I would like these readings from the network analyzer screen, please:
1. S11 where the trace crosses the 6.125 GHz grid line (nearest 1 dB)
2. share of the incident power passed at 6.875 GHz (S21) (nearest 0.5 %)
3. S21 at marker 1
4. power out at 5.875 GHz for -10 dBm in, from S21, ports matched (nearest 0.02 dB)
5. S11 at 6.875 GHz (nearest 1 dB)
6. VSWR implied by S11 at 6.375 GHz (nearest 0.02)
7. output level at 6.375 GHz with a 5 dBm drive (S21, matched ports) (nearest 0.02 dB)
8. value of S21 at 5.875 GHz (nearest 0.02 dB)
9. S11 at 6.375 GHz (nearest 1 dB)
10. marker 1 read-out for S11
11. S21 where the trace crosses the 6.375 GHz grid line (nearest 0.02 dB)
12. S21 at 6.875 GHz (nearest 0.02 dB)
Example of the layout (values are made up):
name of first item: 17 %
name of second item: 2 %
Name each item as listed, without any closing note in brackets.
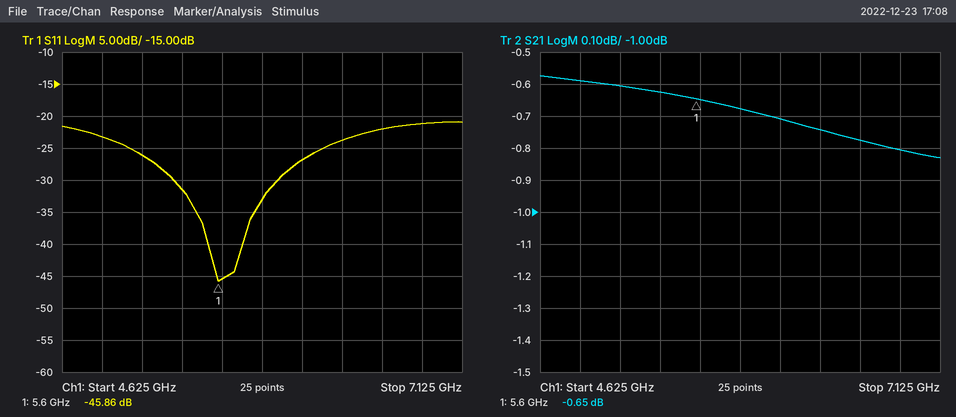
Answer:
S11 where the trace crosses the 6.125 GHz grid line: -27 dB
share of the incident power passed at 6.875 GHz (S21): 83.0 %
S21 at marker 1: -0.65 dB
power out at 5.875 GHz for -10 dBm in, from S21, ports matched: -10.68 dBm
S11 at 6.875 GHz: -21 dB
VSWR implied by S11 at 6.375 GHz: 1.14
output level at 6.375 GHz with a 5 dBm drive (S21, matched ports): 4.26 dBm
value of S21 at 5.875 GHz: -0.68 dB
S11 at 6.375 GHz: -24 dB
marker 1 read-out for S11: -45.86 dB
S21 where the trace crosses the 6.375 GHz grid line: -0.74 dB
S21 at 6.875 GHz: -0.80 dB
